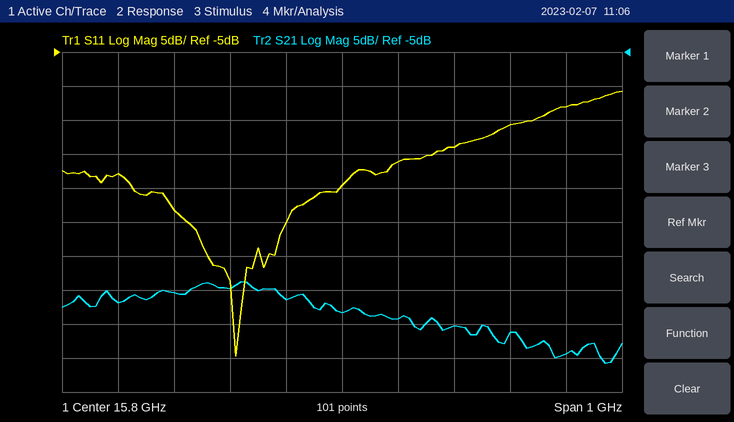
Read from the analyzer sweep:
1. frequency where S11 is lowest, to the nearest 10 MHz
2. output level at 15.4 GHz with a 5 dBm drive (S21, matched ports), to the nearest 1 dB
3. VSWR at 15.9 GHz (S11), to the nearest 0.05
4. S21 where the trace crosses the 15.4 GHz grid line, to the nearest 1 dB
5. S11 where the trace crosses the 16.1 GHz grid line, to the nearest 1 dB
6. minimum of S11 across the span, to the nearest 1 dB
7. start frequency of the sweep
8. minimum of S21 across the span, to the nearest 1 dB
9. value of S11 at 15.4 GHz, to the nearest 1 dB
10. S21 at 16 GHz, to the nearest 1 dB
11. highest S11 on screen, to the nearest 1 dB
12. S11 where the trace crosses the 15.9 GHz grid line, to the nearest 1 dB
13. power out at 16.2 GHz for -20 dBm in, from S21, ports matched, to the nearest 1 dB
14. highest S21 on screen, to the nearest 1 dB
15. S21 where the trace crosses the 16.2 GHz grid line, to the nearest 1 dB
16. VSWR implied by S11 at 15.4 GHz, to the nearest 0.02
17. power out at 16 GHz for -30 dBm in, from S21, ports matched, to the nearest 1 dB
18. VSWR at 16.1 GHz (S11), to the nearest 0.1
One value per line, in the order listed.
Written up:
15.61 GHz
-37 dBm
1.20
-42 dB
-16 dB
-50 dB
15.3 GHz
-51 dB
-23 dB
-45 dB
-11 dB
-21 dB
-69 dBm
-39 dB
-49 dB
1.16
-75 dBm
1.4
